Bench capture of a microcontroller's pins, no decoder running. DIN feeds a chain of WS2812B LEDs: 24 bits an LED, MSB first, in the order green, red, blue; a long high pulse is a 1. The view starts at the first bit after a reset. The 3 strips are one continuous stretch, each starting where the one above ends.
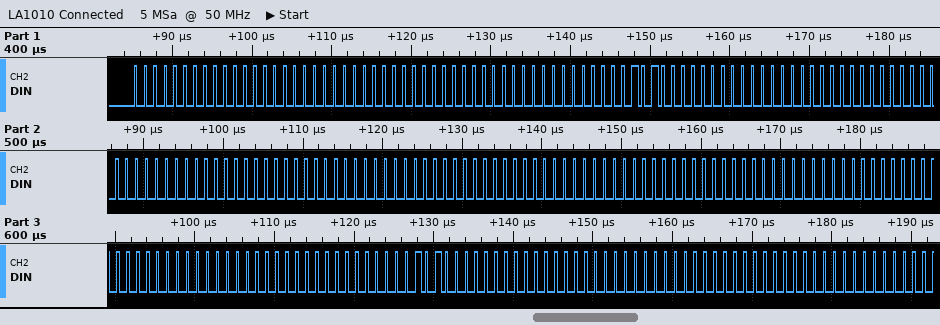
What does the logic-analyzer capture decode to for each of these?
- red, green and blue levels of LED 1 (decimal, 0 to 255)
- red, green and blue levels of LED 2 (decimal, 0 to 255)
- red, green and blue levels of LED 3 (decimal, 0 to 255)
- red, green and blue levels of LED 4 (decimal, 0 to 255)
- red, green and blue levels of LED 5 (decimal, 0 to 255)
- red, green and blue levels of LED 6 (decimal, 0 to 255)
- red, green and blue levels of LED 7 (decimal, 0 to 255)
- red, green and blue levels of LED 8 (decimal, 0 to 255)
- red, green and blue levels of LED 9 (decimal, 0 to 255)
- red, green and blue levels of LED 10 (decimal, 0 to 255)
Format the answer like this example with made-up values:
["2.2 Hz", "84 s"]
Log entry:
["0, 0, 0", "0, 0, 0", "0, 40, 0", "0, 0, 0", "0, 0, 0", "0, 0, 0", "0, 0, 0", "0, 0, 0", "0, 40, 0", "0, 0, 0"]
